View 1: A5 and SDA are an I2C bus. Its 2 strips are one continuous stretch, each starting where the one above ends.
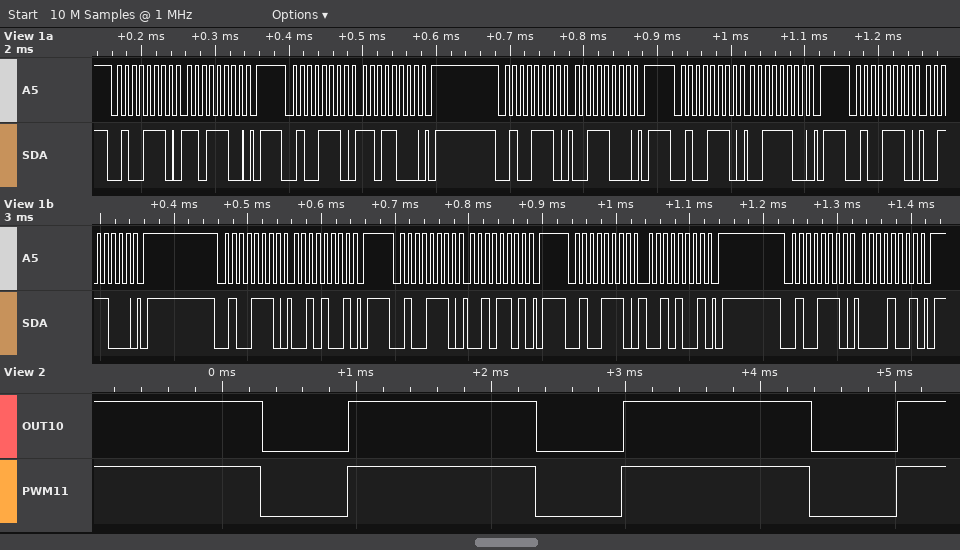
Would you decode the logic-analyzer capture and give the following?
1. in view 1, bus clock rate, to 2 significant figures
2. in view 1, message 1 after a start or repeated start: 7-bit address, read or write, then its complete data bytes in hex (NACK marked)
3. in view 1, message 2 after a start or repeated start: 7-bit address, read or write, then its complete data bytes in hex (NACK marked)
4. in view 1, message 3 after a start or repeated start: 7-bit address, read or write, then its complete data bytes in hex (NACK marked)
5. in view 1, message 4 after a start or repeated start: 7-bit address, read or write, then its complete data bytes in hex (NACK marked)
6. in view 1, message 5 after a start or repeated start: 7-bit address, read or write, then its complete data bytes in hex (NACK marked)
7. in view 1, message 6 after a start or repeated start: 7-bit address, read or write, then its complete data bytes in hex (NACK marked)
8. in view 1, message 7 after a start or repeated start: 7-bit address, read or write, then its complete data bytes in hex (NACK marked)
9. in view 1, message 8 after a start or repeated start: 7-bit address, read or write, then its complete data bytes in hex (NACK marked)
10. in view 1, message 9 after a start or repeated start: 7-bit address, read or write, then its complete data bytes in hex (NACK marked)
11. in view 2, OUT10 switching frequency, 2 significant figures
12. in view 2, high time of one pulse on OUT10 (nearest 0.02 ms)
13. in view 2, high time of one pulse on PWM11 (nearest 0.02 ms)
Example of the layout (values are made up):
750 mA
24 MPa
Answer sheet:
100 kHz
0x27 write: DC
0x27 write: D8
0x27 write: 38
0x27 write: 3C
0x27 write: 38
0x27 write: 29
0x27 write: 2D
0x27 write: 29
0x27 write: 09
490 Hz
1.40 ms
1.40 ms
